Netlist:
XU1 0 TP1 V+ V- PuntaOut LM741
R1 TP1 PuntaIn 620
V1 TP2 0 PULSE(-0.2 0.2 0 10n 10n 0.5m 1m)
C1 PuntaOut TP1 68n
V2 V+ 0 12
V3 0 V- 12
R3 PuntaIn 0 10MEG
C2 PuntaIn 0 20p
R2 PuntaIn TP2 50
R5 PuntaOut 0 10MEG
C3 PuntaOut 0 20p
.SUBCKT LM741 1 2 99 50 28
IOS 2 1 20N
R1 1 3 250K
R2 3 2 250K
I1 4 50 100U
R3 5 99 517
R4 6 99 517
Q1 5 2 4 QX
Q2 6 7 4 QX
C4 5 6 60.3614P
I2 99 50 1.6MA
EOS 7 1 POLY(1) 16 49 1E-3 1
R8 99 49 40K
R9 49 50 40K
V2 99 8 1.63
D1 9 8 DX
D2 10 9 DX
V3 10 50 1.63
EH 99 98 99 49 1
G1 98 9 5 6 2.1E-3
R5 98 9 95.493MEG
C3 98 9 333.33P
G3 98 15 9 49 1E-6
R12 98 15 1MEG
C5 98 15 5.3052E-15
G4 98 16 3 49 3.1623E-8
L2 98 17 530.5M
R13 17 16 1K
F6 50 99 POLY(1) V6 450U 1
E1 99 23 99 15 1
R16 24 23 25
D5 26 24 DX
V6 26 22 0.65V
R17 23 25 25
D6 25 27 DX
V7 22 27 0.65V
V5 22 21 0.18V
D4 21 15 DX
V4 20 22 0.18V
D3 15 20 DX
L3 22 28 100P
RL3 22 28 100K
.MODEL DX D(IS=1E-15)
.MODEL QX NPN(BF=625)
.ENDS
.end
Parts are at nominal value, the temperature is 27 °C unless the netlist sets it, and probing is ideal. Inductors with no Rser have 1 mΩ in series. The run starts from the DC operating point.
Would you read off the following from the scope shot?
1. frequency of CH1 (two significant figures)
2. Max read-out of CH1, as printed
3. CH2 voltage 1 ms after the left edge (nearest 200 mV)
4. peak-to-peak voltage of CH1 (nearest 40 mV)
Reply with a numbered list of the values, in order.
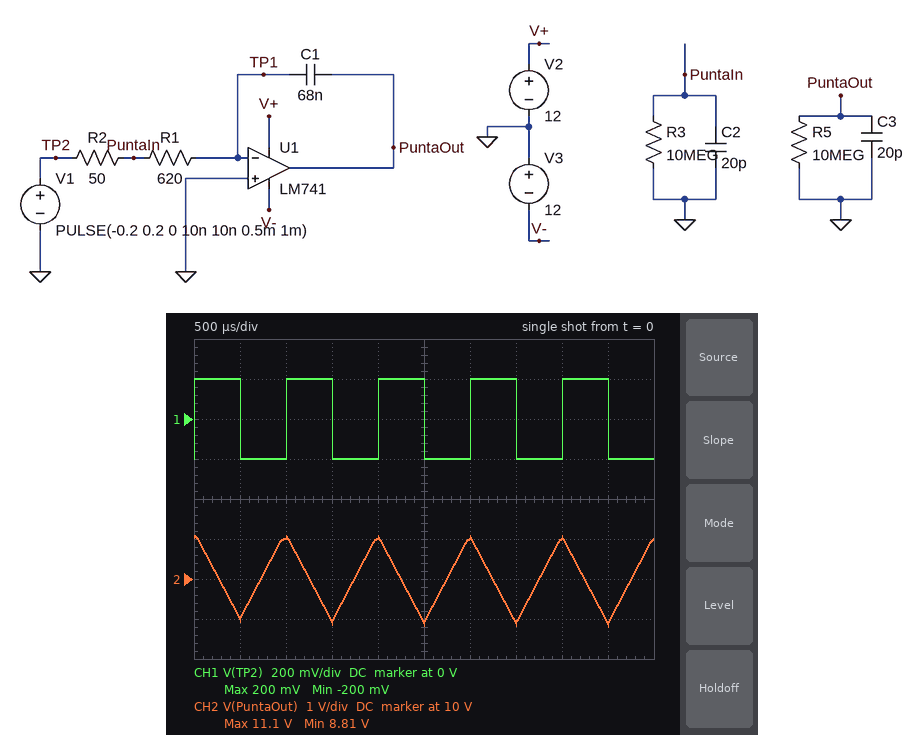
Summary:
1. 1.0 kHz
2. 200 mV
3. 11.0 V
4. 400 mV
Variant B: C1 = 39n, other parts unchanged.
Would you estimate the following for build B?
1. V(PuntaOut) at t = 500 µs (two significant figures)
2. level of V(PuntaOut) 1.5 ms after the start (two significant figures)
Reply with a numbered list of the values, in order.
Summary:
1. 7.4 V
2. 7.3 V
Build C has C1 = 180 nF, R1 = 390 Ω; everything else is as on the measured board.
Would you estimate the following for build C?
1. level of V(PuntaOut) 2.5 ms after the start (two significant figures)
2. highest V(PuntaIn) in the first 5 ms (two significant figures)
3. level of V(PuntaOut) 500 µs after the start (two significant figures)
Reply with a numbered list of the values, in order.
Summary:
1. 9.8 V
2. 180 mV
3. 9.9 V
